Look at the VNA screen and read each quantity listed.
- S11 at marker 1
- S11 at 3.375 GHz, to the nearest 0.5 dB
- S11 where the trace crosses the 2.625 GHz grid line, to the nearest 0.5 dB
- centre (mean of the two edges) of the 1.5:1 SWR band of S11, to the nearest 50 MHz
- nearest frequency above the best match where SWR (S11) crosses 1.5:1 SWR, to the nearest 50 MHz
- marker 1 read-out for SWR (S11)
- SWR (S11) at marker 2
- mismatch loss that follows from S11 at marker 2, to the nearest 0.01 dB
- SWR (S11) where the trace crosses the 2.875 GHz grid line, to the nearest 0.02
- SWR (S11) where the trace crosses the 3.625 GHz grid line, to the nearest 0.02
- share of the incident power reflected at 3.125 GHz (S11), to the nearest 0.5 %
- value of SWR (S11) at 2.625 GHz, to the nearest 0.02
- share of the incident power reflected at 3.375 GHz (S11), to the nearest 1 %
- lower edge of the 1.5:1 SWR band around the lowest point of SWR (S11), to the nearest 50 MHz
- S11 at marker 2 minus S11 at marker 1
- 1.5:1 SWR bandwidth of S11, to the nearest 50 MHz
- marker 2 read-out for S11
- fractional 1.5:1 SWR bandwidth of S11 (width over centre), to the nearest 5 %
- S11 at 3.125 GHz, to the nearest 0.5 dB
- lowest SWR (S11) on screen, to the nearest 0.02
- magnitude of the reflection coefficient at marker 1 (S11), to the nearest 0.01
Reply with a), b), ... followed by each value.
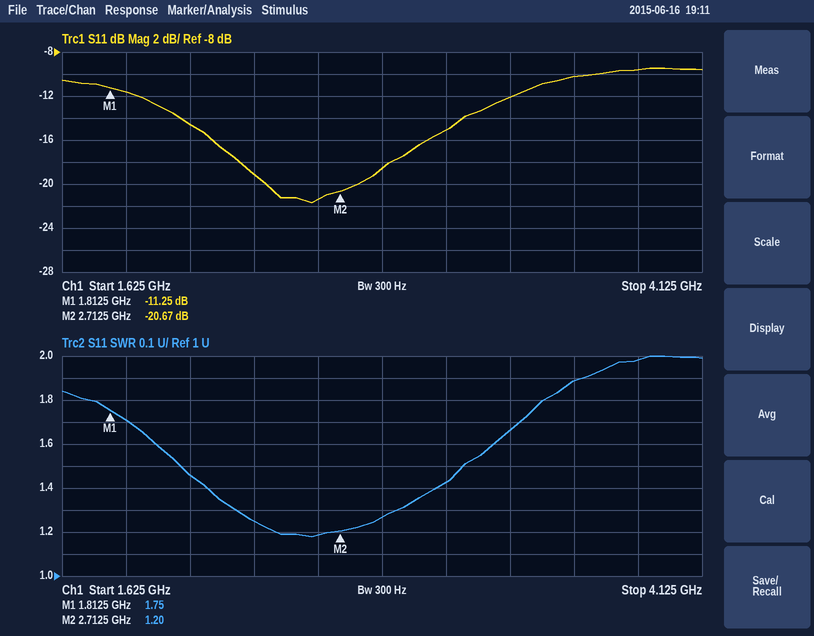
a) -11.25 dB
b) -12.0 dB
c) -21.5 dB
d) 2.65 GHz
e) 3.20 GHz
f) 1.75
g) 1.20
h) 0.04 dB
i) 1.26
j) 1.88
k) 3.0 %
l) 1.18
m) 6 %
n) 2.10 GHz
o) -9.42 dB
p) 1.10 GHz
q) -20.67 dB
r) 40 %
s) -15.0 dB
t) 1.18
u) 0.27
